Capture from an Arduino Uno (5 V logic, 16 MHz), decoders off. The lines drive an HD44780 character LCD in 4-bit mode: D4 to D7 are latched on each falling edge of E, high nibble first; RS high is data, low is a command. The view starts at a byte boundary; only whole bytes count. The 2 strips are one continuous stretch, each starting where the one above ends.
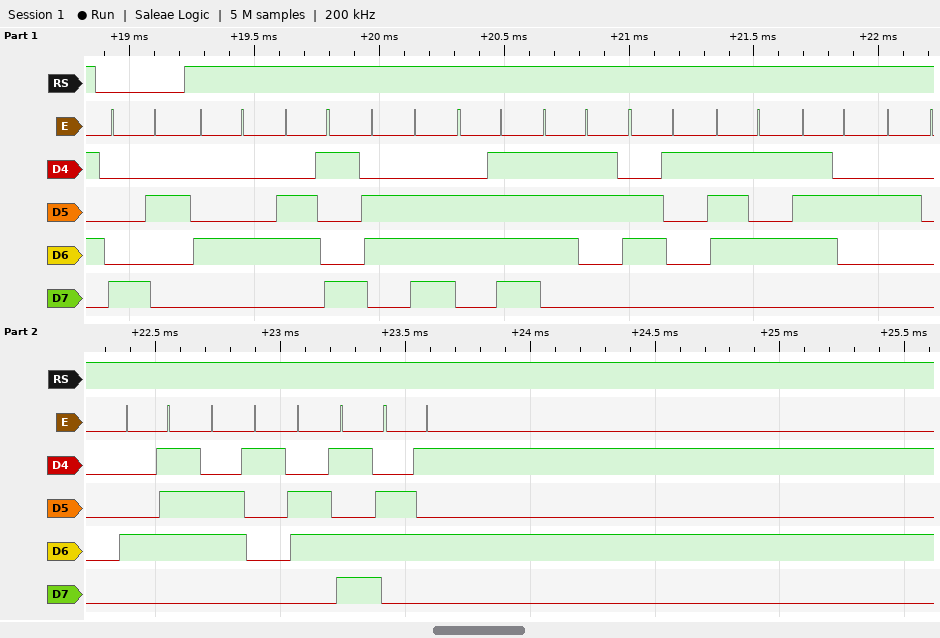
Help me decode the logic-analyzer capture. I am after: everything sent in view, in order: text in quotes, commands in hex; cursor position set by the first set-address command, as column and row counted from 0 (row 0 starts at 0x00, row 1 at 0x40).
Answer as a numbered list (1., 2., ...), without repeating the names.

1. 0x82 "Dinosaur Game"
2. column 2, row 0
